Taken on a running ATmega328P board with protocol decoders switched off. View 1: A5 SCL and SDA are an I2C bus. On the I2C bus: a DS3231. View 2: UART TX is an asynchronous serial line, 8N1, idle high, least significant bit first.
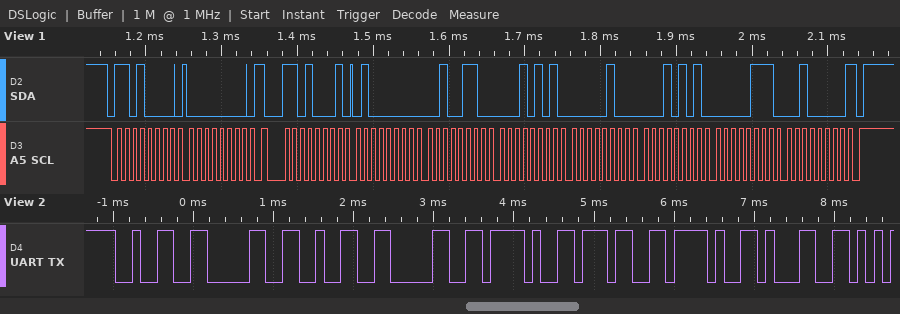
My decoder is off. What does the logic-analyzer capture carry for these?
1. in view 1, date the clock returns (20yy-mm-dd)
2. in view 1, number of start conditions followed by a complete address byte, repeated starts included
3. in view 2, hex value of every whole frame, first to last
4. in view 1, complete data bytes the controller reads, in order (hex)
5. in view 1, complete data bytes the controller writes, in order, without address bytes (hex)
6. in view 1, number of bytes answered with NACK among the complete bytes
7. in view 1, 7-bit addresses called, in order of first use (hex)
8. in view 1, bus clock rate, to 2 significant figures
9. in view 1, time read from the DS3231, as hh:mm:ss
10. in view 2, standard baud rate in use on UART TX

2020-07-15
2
32 30 32 30 2F 37 2F 31
40 26 15 04 15 07 20
00
1
0x68
100 kHz
15:26:40
9600 baud
